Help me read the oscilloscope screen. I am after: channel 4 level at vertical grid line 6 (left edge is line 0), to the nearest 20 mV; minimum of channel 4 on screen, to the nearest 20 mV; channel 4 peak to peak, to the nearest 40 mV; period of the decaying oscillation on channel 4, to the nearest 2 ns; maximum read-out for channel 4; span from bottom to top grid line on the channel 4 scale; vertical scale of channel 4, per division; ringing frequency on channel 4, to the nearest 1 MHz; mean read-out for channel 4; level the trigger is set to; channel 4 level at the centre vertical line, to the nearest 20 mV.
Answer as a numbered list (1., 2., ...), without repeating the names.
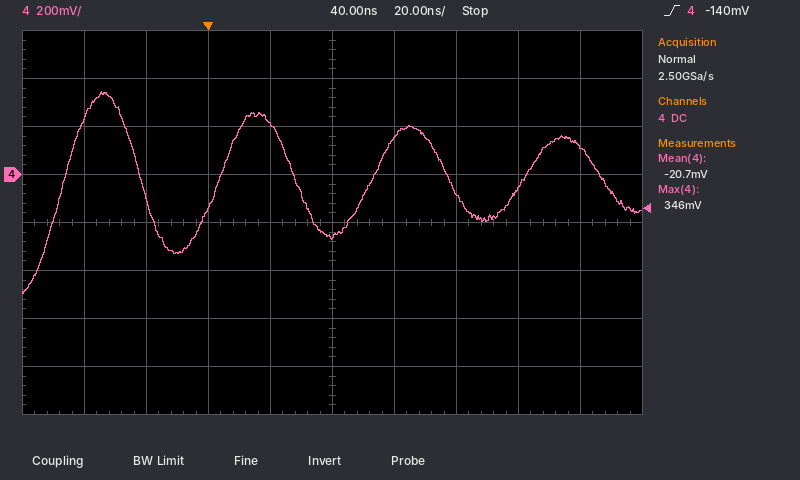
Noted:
1. 160 mV
2. -500 mV
3. 840 mV
4. 50 ns
5. 346 mV
6. 1.6 V
7. 200 mV
8. 20 MHz
9. -20.7 mV
10. -140 mV
11. -260 mV
